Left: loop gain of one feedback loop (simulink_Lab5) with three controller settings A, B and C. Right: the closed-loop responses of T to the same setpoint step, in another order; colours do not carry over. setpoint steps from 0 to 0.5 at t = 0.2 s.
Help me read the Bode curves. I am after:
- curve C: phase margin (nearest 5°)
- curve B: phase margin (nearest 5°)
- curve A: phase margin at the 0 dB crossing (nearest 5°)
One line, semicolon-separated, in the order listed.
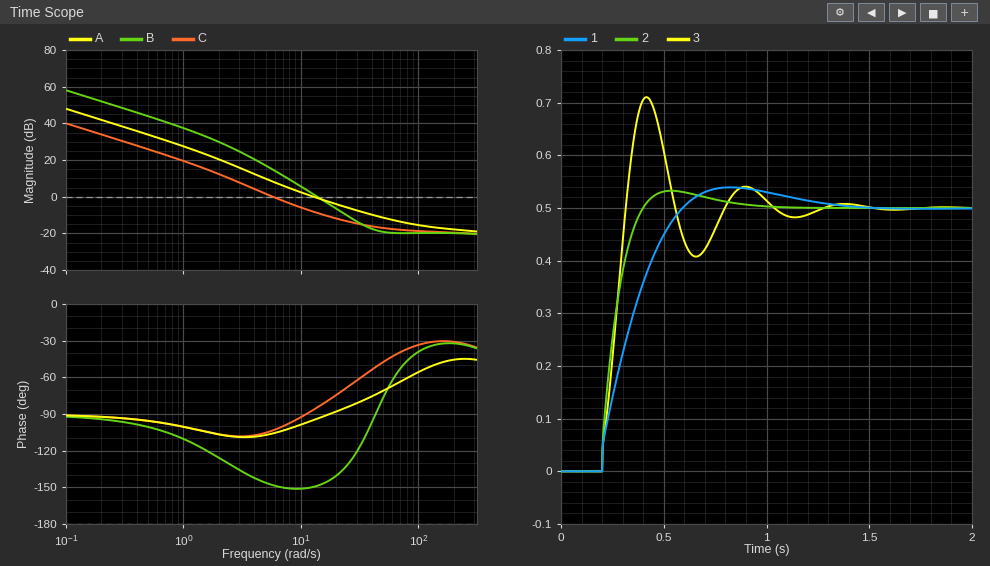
75°; 30°; 85°
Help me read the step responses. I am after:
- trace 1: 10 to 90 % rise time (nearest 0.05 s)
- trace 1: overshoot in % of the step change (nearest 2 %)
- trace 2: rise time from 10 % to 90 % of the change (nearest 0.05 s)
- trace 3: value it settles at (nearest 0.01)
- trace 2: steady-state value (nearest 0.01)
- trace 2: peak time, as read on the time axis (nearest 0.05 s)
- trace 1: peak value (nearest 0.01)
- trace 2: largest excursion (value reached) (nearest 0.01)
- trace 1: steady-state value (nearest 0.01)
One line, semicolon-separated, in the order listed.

0.30 s; 8 %; 0.15 s; 0.50; 0.50; 0.55 s; 0.54; 0.53; 0.50
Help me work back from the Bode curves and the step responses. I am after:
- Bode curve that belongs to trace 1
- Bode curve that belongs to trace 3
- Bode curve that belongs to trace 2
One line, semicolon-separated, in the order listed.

C; B; A
